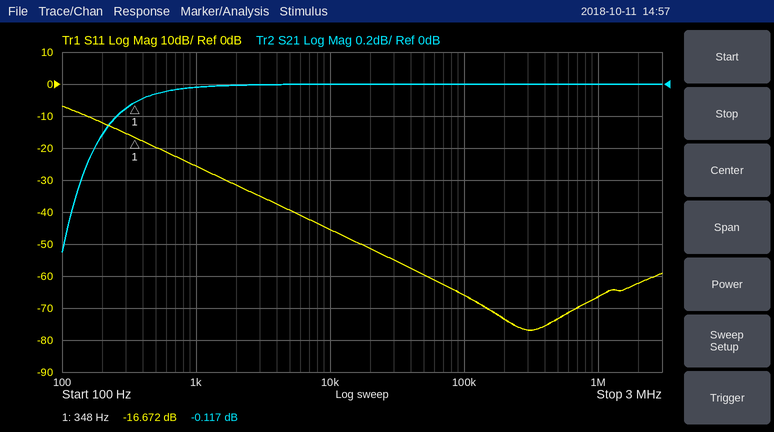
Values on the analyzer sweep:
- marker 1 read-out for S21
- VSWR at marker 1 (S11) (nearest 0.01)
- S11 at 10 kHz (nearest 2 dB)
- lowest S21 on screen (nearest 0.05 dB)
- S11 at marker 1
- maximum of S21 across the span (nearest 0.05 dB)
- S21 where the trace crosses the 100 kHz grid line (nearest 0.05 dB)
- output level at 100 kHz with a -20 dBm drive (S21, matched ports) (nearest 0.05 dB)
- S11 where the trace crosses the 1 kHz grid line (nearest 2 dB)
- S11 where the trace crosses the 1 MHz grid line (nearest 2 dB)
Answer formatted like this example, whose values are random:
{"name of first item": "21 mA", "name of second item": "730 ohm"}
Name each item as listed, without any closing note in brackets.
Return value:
{"marker 1 read-out for S21": "-0.117 dB", "VSWR at marker 1 (S11)": "1.34", "S11 at 10 kHz": "-46 dB", "lowest S21 on screen": "-1.05 dB", "S11 at marker 1": "-16.672 dB", "maximum of S21 across the span": "0.00 dB", "S21 where the trace crosses the 100 kHz grid line": "0.00 dB", "output level at 100 kHz with a -20 dBm drive (S21, matched ports)": "-20.00 dBm", "S11 where the trace crosses the 1 kHz grid line": "-26 dB", "S11 where the trace crosses the 1 MHz grid line": "-66 dB"}
